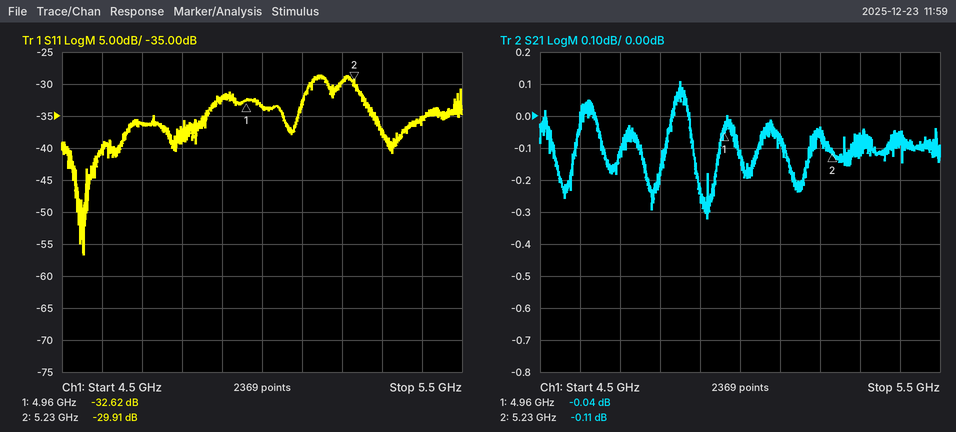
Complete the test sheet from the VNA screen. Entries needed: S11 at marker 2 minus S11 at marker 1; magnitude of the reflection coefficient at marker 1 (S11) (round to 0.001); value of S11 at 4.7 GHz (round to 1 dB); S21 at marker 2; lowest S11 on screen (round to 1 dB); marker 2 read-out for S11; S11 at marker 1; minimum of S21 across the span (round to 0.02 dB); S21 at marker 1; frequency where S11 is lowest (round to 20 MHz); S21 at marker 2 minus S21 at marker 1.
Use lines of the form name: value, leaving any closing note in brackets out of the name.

S11 at marker 2 minus S11 at marker 1: 2.71 dB
magnitude of the reflection coefficient at marker 1 (S11): 0.023
value of S11 at 4.7 GHz: -36 dB
S21 at marker 2: -0.11 dB
lowest S11 on screen: -57 dB
marker 2 read-out for S11: -29.91 dB
S11 at marker 1: -32.62 dB
minimum of S21 across the span: -0.32 dB
S21 at marker 1: -0.04 dB
frequency where S11 is lowest: 4.56 GHz
S21 at marker 2 minus S21 at marker 1: -0.07 dB
